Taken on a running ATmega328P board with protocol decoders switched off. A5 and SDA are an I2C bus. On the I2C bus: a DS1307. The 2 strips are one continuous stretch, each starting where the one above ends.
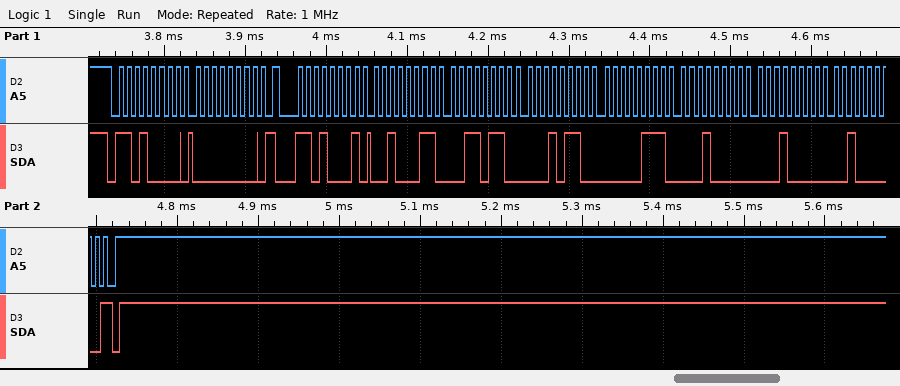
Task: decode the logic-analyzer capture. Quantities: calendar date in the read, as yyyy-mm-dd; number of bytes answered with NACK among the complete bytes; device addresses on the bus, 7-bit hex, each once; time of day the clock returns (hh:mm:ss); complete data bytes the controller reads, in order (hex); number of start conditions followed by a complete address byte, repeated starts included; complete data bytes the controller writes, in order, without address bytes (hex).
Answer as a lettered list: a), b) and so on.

a) 2020-10-10
b) 1
c) 0x68
d) 16:36:23
e) 23 36 16 07 10 10 20
f) 2
g) 00
